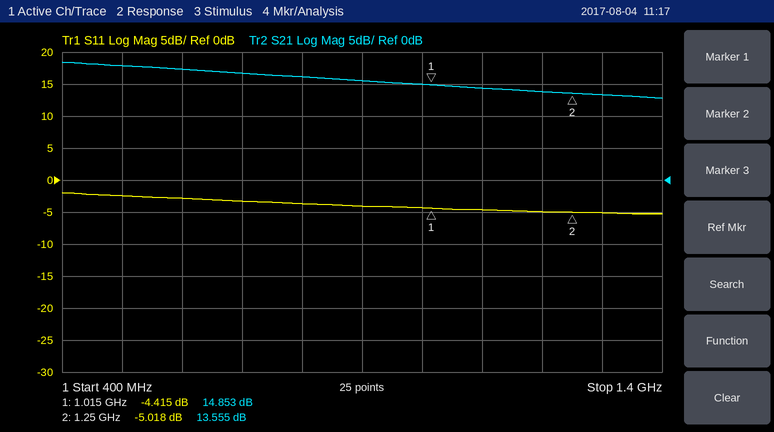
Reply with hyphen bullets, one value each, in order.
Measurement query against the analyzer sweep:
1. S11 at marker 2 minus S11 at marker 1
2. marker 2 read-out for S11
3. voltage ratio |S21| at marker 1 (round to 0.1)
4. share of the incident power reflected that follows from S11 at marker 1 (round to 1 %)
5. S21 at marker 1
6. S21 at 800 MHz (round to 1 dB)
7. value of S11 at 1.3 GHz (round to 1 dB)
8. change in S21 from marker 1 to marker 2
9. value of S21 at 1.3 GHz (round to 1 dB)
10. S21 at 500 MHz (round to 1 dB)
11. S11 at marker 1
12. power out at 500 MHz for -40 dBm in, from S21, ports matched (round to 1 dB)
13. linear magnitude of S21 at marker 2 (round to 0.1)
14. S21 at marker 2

- -0.603 dB
- -5.018 dB
- 5.5
- 36 %
- 14.853 dB
- 16 dB
- -5 dB
- -1.298 dB
- 13 dB
- 18 dB
- -4.415 dB
- -22 dBm
- 4.8
- 13.555 dB
